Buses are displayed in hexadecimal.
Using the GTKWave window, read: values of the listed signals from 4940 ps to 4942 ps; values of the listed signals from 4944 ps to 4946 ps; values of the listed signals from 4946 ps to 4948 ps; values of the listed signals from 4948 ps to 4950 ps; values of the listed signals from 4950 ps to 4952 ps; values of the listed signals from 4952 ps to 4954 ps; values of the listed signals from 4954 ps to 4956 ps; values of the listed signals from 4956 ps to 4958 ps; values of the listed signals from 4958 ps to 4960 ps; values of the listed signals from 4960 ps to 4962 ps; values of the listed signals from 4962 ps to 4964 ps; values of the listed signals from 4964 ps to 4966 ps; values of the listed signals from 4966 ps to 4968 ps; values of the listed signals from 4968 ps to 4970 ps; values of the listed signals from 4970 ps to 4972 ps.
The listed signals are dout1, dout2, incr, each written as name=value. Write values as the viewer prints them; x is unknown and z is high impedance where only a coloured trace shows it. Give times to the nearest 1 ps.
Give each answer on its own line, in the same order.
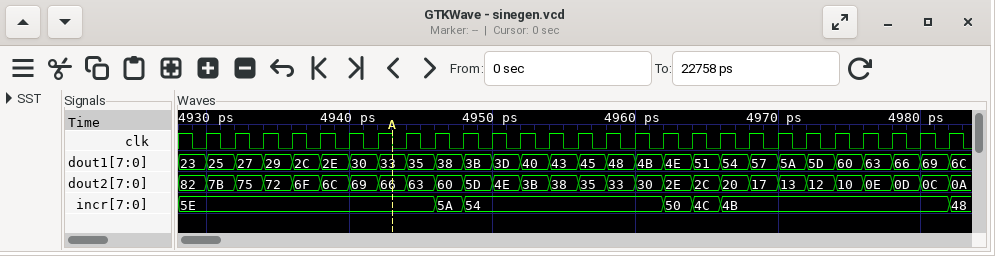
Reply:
dout1=30, dout2=69, incr=5E
dout1=35, dout2=63, incr=5E
dout1=38, dout2=60, incr=5A
dout1=3B, dout2=5D, incr=54
dout1=3D, dout2=4E, incr=54
dout1=40, dout2=3B, incr=54
dout1=43, dout2=38, incr=54
dout1=45, dout2=35, incr=54
dout1=48, dout2=33, incr=54
dout1=4B, dout2=30, incr=54
dout1=4E, dout2=2E, incr=50
dout1=51, dout2=2C, incr=4C
dout1=54, dout2=20, incr=4B
dout1=57, dout2=17, incr=4B
dout1=5A, dout2=13, incr=4B
